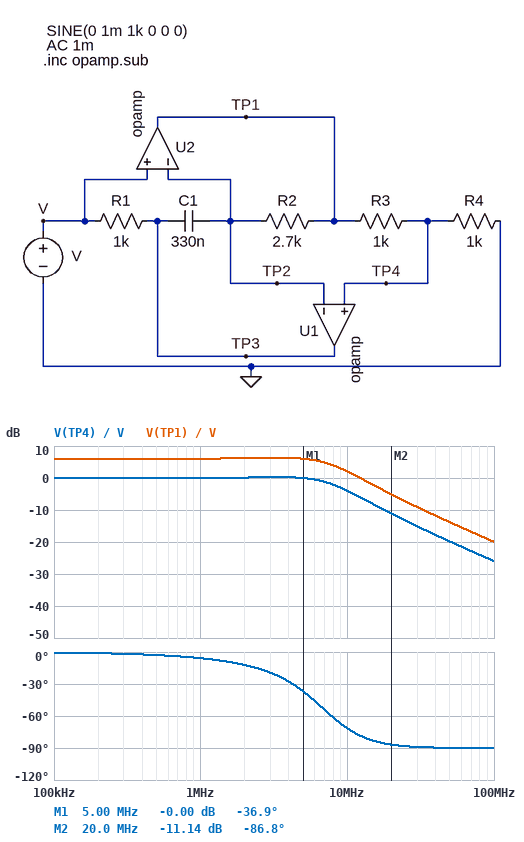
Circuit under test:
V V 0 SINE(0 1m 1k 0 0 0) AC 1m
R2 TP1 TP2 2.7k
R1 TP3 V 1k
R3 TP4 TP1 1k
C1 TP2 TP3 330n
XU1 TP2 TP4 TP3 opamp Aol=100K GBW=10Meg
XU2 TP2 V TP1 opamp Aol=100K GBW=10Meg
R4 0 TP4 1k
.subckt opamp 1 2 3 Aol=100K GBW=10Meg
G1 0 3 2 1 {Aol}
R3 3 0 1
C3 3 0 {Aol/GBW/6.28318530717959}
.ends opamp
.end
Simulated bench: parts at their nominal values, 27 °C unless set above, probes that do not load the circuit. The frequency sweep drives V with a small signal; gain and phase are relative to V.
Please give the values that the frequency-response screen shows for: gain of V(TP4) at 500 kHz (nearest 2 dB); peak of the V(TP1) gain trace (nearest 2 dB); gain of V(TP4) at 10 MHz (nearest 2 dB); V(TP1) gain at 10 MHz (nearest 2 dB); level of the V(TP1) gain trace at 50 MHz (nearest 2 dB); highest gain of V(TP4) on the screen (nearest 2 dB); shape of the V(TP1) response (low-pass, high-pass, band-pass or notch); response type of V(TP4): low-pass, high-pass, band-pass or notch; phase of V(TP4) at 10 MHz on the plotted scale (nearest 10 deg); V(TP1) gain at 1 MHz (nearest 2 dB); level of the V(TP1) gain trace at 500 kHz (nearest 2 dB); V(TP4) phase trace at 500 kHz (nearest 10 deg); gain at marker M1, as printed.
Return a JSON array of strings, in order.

["0 dB", "6 dB", "-4 dB", "2 dB", "-14 dB", "0 dB", "low-pass", "low-pass", "-70 deg", "6 dB", "6 dB", "0 deg", "-0.00 dB"]
